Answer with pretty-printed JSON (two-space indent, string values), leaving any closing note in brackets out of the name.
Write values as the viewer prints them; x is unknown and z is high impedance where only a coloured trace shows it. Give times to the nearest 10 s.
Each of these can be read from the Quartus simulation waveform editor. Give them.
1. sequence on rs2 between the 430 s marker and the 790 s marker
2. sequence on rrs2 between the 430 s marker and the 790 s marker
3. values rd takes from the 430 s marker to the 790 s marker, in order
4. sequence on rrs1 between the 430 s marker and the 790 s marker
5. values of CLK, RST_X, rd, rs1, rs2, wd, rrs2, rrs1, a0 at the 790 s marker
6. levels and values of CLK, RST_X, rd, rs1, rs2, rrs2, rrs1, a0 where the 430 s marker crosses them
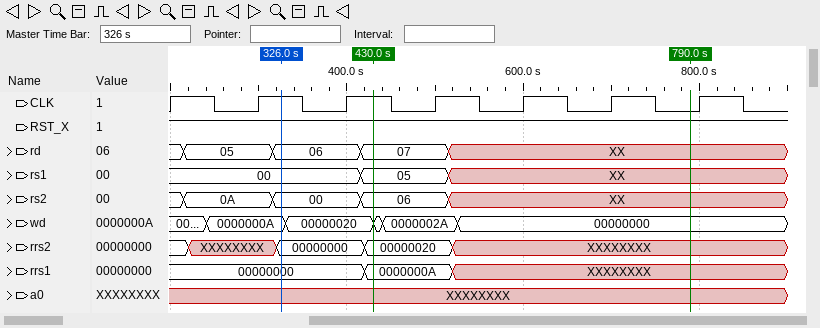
{
  "sequence on rs2 between the 430 s marker and the 790 s marker": "06, XX",
  "sequence on rrs2 between the 430 s marker and the 790 s marker": "00000020, XXXXXXXX",
  "values rd takes from the 430 s marker to the 790 s marker, in order": "07, XX",
  "sequence on rrs1 between the 430 s marker and the 790 s marker": "0000000A, XXXXXXXX",
  "values of CLK, RST_X, rd, rs1, rs2, wd, rrs2, rrs1, a0 at the 790 s marker": "CLK=0, RST_X=1, rd=XX, rs1=XX, rs2=XX, wd=00000000, rrs2=XXXXXXXX, rrs1=XXXXXXXX, a0=XXXXXXXX",
  "levels and values of CLK, RST_X, rd, rs1, rs2, rrs2, rrs1, a0 where the 430 s marker crosses them": "CLK=1, RST_X=1, rd=07, rs1=05, rs2=06, rrs2=00000020, rrs1=0000000A, a0=XXXXXXXX"
}
